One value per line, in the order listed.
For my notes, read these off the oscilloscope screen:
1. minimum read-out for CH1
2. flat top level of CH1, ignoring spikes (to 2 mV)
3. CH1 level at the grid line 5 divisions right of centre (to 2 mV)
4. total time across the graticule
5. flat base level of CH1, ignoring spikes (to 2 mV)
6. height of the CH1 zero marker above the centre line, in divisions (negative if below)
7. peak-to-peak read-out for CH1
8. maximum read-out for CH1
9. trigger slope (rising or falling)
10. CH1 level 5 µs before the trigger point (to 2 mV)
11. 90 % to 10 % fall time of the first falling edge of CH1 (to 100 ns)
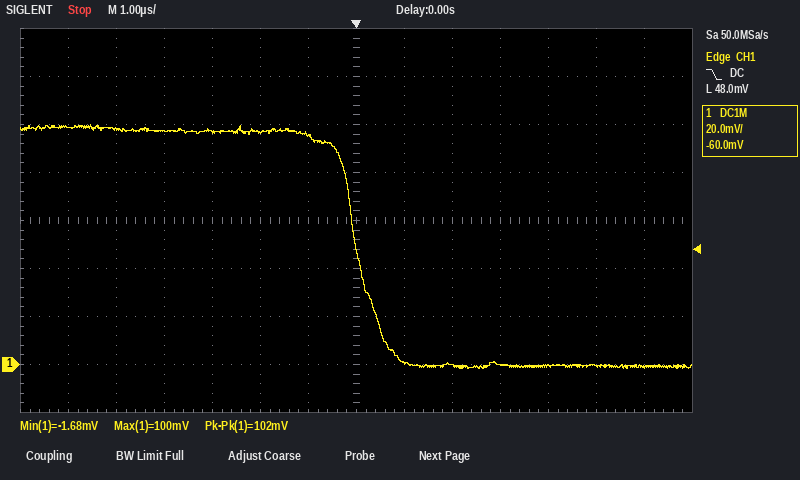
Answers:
-1.68 mV
98 mV
0 mV
14 µs
0 mV
-3.0 div
102 mV
100 mV
falling
98 mV
1.0 µs
